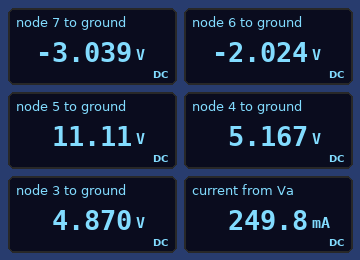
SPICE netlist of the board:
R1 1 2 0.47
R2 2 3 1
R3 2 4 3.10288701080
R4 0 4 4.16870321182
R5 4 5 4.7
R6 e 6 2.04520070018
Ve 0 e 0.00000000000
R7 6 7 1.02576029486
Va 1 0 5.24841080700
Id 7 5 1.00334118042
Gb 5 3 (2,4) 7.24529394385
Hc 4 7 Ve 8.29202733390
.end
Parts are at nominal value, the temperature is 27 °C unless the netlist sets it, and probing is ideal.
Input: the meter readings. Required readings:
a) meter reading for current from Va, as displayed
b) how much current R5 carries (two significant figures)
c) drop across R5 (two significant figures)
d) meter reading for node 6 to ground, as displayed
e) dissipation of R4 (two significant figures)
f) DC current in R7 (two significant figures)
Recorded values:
249.8 mA
1.3 A
5.9 V
-2.024 V
6.4 W
990 mA
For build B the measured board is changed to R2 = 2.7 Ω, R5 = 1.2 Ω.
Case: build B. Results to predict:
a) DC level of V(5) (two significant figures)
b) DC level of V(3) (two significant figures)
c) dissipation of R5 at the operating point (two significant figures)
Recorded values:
6.7 V
4.4 V
1.9 W
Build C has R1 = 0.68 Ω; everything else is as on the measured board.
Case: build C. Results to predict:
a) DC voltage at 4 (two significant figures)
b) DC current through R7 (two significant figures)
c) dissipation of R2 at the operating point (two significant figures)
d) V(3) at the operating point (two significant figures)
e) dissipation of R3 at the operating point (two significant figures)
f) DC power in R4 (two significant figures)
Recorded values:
5.1 V
980 mA
67 mW
4.8 V
410 µW
6.3 W
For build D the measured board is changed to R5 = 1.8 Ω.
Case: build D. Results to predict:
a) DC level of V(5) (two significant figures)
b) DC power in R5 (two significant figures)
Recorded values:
7.4 V
2.9 W
